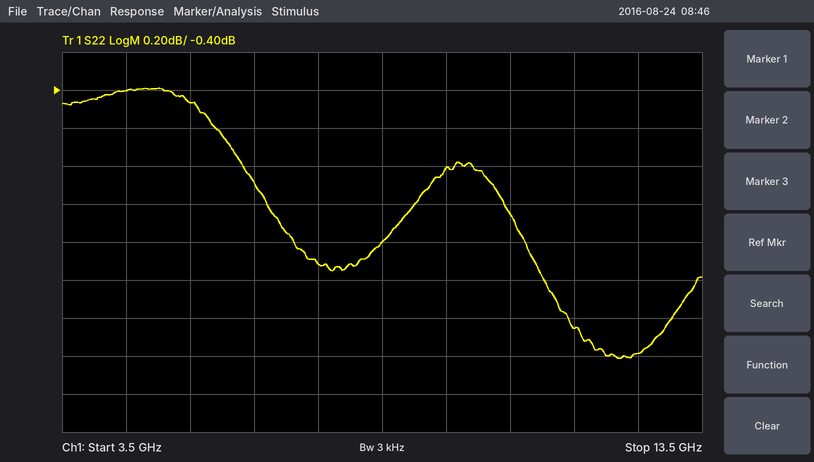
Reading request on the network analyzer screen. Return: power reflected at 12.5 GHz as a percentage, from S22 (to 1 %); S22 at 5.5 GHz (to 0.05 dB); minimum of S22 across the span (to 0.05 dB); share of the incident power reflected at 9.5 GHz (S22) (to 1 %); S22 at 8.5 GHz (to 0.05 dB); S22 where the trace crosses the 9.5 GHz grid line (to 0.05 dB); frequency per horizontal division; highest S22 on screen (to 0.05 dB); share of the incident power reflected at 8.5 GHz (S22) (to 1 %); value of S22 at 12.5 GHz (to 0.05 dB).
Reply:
66 %
-0.45 dB
-1.80 dB
83 %
-1.20 dB
-0.80 dB
1 GHz
-0.40 dB
76 %
-1.80 dB
